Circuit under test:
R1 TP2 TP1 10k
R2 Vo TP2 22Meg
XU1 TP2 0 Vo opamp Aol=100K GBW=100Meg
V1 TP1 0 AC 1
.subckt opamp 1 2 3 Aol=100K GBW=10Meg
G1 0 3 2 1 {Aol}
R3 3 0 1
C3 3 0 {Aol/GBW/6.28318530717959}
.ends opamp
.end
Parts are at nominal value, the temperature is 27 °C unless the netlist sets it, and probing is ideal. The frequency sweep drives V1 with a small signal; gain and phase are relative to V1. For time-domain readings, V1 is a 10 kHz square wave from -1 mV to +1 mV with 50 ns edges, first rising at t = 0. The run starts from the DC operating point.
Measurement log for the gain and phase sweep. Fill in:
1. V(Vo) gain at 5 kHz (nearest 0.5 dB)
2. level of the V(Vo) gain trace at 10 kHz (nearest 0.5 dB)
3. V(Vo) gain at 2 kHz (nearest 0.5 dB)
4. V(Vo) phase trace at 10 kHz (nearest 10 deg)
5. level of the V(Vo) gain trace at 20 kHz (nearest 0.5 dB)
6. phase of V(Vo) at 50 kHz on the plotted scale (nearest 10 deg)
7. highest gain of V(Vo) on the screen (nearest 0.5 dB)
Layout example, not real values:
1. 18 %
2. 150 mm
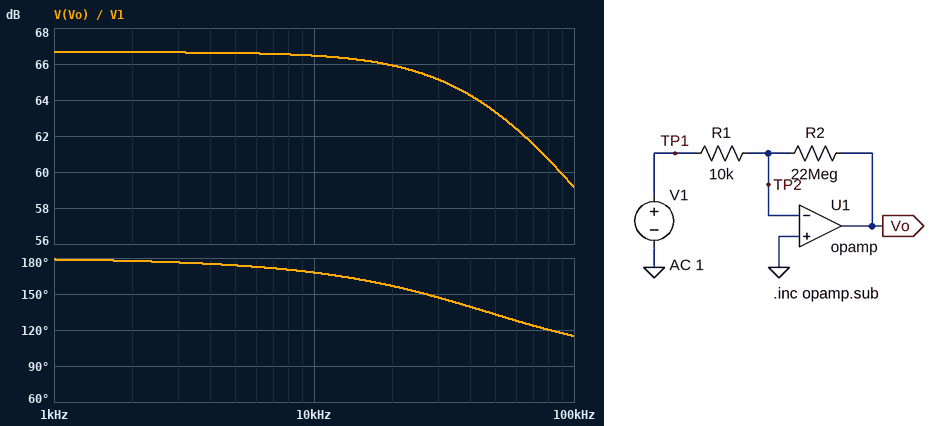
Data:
1. 66.5 dB
2. 66.5 dB
3. 66.5 dB
4. 170 deg
5. 66.0 dB
6. 130 deg
7. 66.5 dB
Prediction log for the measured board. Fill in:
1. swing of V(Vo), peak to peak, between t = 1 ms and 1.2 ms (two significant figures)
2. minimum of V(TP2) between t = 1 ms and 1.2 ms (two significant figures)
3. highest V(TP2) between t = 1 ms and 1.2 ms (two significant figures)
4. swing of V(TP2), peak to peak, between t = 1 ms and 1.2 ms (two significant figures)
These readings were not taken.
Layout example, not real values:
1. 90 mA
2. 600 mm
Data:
1. 4.3 V
2. -2.0 mV
3. 2.0 mV
4. 3.9 mV
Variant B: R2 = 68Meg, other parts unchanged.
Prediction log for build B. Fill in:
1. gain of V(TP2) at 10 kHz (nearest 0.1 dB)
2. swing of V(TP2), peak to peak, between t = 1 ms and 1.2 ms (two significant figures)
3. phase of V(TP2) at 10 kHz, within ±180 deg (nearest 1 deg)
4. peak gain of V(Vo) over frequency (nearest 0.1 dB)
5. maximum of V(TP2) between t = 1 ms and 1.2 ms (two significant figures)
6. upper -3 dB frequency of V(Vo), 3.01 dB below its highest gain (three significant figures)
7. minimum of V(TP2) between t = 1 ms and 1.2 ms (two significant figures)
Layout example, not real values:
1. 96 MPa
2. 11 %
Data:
1. -5.4 dB
2. 3.8 mV
3. 52 deg
4. 76.1 dB
5. 1.9 mV
6. 15.7 kHz
7. -1.9 mV
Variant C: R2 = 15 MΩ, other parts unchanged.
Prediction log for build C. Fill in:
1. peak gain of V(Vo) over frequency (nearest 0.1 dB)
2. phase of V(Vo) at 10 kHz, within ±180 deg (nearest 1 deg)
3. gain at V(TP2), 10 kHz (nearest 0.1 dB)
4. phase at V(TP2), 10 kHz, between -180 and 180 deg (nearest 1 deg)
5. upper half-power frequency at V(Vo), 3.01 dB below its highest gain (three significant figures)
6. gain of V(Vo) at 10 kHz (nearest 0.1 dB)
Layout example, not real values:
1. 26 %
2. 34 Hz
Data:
1. 63.4 dB
2. 172 deg
3. -16.7 dB
4. 76 deg
5. 67.6 kHz
6. 63.3 dB
